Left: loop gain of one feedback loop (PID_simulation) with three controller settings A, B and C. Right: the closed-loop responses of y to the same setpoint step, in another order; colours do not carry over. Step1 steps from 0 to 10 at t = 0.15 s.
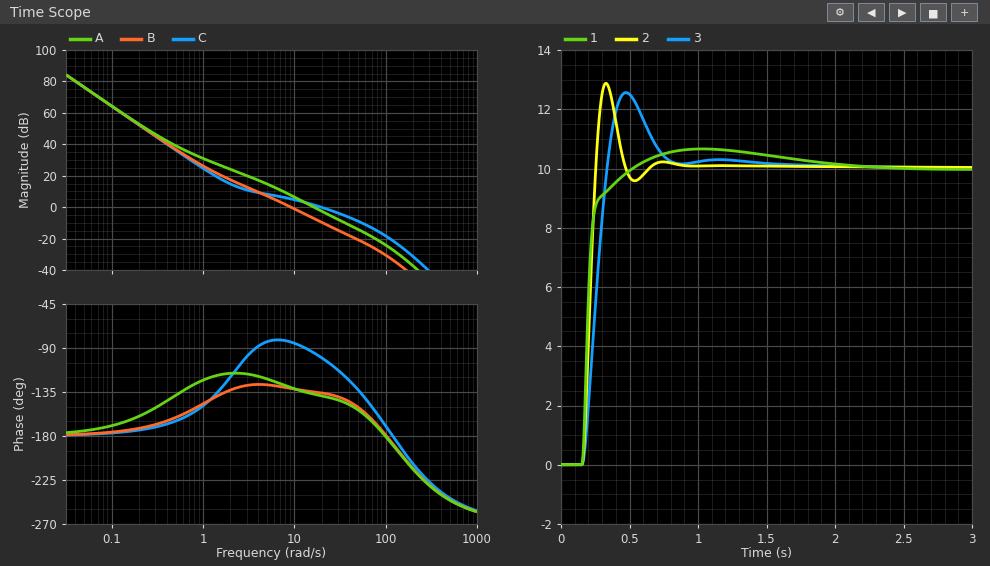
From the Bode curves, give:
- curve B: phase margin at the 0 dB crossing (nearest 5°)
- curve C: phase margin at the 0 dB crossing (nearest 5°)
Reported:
50°
80°
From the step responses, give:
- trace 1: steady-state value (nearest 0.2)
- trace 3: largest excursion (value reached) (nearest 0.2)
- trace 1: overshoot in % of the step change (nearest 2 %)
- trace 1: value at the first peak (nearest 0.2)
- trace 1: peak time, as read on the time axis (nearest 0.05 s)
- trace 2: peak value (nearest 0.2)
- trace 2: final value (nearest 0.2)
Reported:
10.0
12.6
6 %
10.6
1.05 s
12.8
10.0
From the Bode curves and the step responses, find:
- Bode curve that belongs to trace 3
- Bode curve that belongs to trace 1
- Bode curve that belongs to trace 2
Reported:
B
C
A
